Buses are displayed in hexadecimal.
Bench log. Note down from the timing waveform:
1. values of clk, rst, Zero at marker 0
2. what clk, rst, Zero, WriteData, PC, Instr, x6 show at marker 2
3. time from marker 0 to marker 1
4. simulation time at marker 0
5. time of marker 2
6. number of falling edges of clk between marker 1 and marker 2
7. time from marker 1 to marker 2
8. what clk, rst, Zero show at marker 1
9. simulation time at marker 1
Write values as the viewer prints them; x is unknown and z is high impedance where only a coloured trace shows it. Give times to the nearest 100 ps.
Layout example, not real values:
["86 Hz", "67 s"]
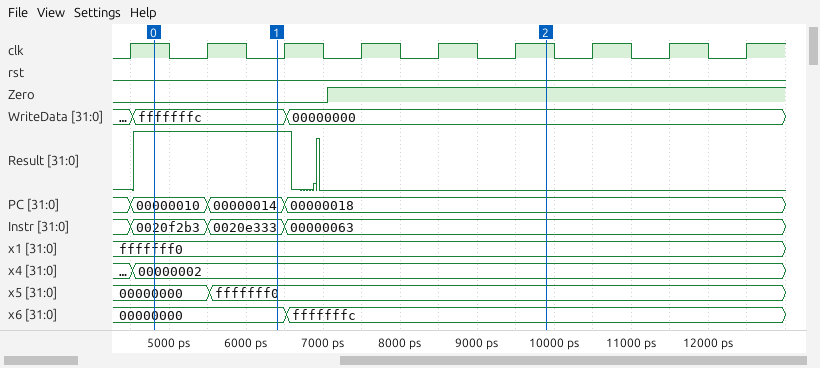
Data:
["clk=1, rst=0, Zero=0", "clk=1, rst=0, Zero=1, WriteData=00000000, PC=00000018, Instr=00000063, x6=fffffffc", "1600 ps", "4800 ps", "9900 ps", "3", "3500 ps", "clk=0, rst=0, Zero=0", "6400 ps"]
